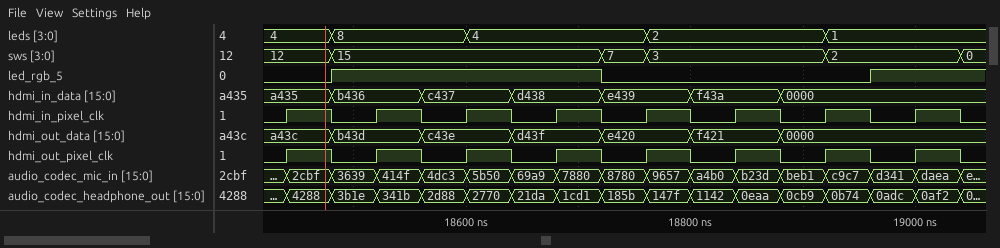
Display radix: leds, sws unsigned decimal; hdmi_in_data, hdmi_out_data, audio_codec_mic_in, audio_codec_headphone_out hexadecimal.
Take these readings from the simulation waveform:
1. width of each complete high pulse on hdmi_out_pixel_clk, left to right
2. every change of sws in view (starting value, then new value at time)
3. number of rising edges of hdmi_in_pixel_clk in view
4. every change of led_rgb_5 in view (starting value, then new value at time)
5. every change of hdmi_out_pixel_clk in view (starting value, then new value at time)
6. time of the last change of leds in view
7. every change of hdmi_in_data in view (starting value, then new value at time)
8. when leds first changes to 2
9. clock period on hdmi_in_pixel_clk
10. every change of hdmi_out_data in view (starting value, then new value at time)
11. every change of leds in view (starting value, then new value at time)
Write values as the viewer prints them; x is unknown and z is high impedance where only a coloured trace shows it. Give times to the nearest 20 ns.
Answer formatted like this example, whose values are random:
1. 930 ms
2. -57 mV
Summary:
1. 40 ns, 40 ns, 40 ns, 40 ns, 40 ns, 40 ns, 40 ns, 40 ns
2. 12, 15 at 18480 ns, 7 at 18720 ns, 3 at 18760 ns, 2 at 18920 ns, 0 at 19040 ns
3. 8
4. 0, 1 at 18480 ns, 0 at 18720 ns, 1 at 18960 ns
5. 0, 1 at 18440 ns, 0 at 18480 ns, 1 at 18520 ns, 0 at 18560 ns, 1 at 18600 ns, 0 at 18640 ns, 1 at 18680 ns, 0 at 18720 ns, 1 at 18760 ns, 0 at 18800 ns, 1 at 18840 ns, 0 at 18880 ns, 1 at 18920 ns, 0 at 18960 ns, 1 at 19000 ns, 0 at 19040 ns
6. 18920 ns
7. a435, b436 at 18480 ns, c437 at 18560 ns, d438 at 18640 ns, e439 at 18720 ns, f43a at 18800 ns, 0000 at 18880 ns
8. 18760 ns
9. 80 ns
10. a43c, b43d at 18480 ns, c43e at 18560 ns, d43f at 18640 ns, e420 at 18720 ns, f421 at 18800 ns, 0000 at 18880 ns
11. 4, 8 at 18480 ns, 4 at 18600 ns, 2 at 18760 ns, 1 at 18920 ns
